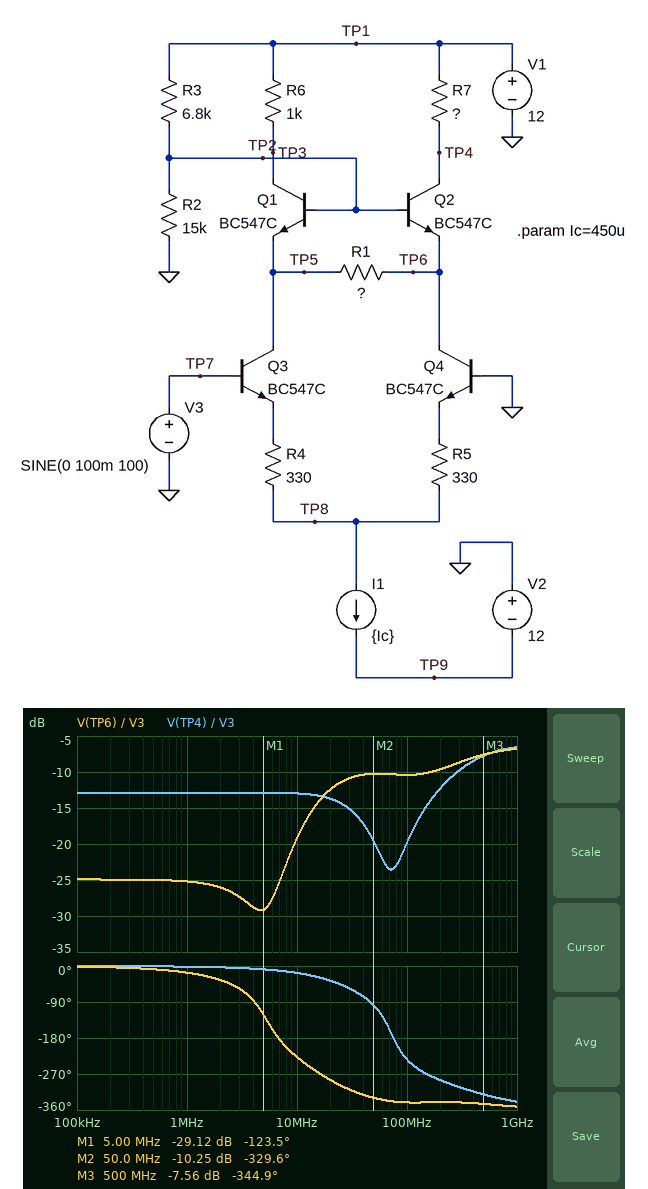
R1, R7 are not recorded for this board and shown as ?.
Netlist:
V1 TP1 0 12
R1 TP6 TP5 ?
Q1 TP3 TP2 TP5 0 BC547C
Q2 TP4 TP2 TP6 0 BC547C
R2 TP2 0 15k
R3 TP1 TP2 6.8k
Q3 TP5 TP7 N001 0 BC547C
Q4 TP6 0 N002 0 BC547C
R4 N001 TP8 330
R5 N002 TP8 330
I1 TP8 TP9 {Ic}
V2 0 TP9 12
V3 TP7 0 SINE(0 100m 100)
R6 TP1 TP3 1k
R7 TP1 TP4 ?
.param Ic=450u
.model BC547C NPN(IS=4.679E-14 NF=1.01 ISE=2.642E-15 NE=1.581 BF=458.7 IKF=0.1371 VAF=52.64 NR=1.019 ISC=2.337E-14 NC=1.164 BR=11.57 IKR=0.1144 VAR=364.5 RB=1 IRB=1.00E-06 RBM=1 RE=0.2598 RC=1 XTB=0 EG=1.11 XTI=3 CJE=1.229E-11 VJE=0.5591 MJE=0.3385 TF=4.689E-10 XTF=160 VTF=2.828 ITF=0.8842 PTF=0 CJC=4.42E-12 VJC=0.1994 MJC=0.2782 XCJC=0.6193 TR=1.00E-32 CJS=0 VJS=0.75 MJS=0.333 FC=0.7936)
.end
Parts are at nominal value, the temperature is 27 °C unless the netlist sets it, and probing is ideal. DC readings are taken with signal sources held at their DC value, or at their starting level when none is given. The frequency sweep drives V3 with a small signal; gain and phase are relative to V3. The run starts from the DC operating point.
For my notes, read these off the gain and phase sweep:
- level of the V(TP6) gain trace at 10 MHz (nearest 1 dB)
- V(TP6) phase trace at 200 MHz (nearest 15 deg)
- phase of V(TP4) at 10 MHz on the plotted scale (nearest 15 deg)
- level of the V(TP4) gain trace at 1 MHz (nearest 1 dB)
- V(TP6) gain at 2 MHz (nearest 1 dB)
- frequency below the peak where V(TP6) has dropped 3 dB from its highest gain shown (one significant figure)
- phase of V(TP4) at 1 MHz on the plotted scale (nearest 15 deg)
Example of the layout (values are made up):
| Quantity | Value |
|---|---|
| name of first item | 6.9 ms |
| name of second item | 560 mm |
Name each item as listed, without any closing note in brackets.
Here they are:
| Quantity | Value |
|---|---|
| level of the V(TP6) gain trace at 10 MHz | -19 dB |
| V(TP6) phase trace at 200 MHz | -345 deg |
| phase of V(TP4) at 10 MHz on the plotted scale | -15 deg |
| level of the V(TP4) gain trace at 1 MHz | -13 dB |
| V(TP6) gain at 2 MHz | -26 dB |
| frequency below the peak where V(TP6) has dropped 3 dB from its highest gain shown | 200 MHz |
| phase of V(TP4) at 1 MHz on the plotted scale | 0 deg |
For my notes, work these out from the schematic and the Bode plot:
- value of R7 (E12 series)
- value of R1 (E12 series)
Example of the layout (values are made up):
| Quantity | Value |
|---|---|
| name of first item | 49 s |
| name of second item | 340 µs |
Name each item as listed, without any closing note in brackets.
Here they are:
| Quantity | Value |
|---|---|
| value of R7 | 470 Ω |
| value of R1 | 180 Ω |
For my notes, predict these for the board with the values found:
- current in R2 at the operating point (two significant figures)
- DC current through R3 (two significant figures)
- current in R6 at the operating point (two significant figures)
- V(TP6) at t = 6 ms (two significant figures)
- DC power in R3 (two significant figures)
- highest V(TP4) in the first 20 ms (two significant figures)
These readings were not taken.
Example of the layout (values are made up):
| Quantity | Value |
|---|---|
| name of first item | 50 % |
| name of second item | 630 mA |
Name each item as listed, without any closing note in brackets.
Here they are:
| Quantity | Value |
|---|---|
| current in R2 at the operating point | 550 µA |
| DC current through R3 | 550 µA |
| current in R6 at the operating point | 220 µA |
| V(TP6) at t = 6 ms | 7.7 V |
| DC power in R3 | 2.1 mW |
| highest V(TP4) in the first 20 ms | 12 V |
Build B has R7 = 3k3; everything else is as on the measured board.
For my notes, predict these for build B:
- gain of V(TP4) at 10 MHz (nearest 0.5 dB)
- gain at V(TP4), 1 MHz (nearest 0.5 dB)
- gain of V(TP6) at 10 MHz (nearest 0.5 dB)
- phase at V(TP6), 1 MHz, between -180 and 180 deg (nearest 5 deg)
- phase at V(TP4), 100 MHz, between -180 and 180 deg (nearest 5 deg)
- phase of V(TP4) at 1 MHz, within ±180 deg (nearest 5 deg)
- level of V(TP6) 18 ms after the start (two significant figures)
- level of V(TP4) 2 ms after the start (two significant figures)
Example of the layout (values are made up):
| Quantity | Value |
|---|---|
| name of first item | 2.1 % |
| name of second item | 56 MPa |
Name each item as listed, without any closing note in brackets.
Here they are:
| Quantity | Value |
|---|---|
| gain of V(TP4) at 10 MHz | 3.0 dB |
| gain at V(TP4), 1 MHz | 4.0 dB |
| gain of V(TP6) at 10 MHz | -7.5 dB |
| phase at V(TP6), 1 MHz, between -180 and 180 deg | 45 deg |
| phase at V(TP4), 100 MHz, between -180 and 180 deg | 80 deg |
| phase of V(TP4) at 1 MHz, within ±180 deg | -5 deg |
| level of V(TP6) 18 ms after the start | 7.7 V |
| level of V(TP4) 2 ms after the start | 11 V |
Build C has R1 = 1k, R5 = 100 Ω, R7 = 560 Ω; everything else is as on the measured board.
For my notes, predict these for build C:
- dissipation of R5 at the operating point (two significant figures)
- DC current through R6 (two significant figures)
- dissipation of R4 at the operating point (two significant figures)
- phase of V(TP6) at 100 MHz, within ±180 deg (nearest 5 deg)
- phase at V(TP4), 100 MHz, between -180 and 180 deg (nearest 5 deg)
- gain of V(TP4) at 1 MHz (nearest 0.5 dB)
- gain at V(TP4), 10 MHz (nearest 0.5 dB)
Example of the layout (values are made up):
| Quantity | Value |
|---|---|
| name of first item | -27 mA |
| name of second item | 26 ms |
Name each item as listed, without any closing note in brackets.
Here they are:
| Quantity | Value |
|---|---|
| dissipation of R5 at the operating point | 9.1 µW |
| DC current through R6 | 160 µA |
| dissipation of R4 at the operating point | 7.2 µW |
| phase of V(TP6) at 100 MHz, within ±180 deg | -15 deg |
| phase at V(TP4), 100 MHz, between -180 and 180 deg | 160 deg |
| gain of V(TP4) at 1 MHz | -4.0 dB |
| gain at V(TP4), 10 MHz | -3.5 dB |
